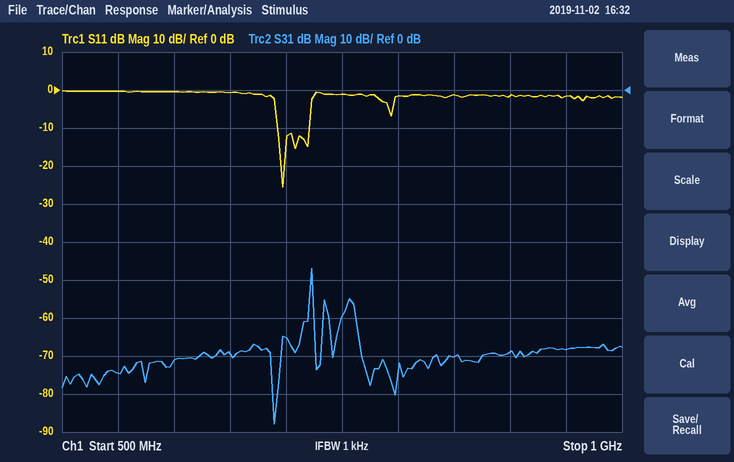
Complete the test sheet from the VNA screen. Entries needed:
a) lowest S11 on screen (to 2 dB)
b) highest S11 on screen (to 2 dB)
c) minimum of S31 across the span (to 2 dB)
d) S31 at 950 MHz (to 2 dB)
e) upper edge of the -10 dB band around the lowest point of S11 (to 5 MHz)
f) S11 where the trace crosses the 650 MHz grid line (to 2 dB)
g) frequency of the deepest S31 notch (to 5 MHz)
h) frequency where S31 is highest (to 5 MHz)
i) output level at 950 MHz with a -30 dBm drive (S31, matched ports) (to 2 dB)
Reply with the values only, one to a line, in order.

-26 dB
0 dB
-88 dB
-68 dB
720 MHz
0 dB
690 MHz
725 MHz
-98 dBm
